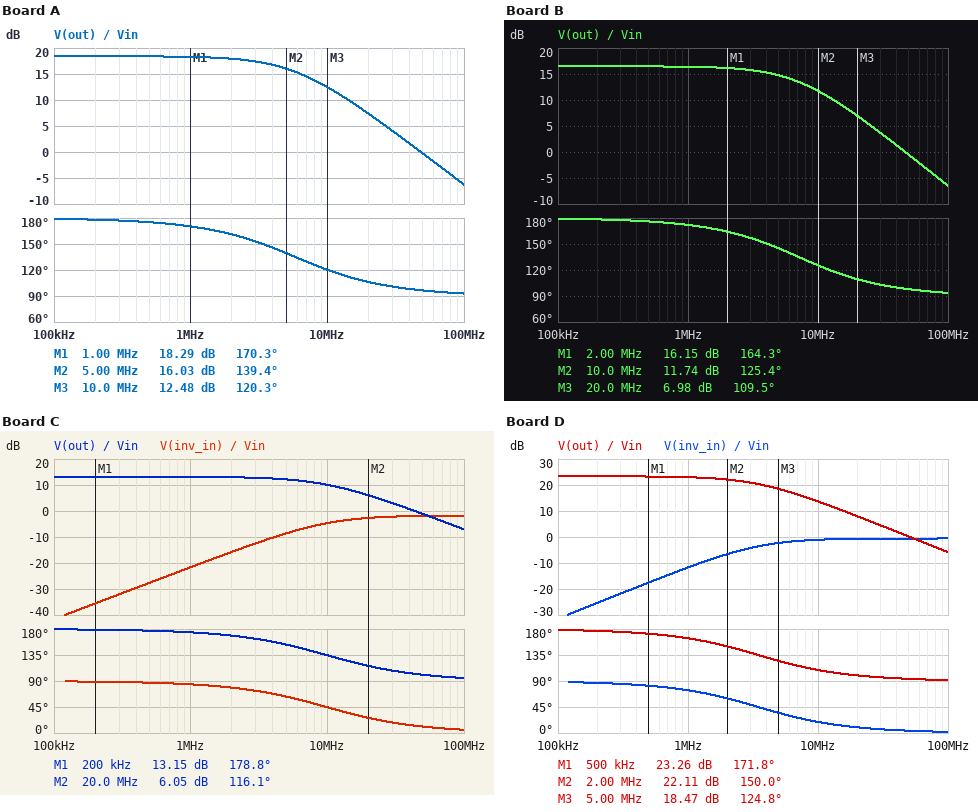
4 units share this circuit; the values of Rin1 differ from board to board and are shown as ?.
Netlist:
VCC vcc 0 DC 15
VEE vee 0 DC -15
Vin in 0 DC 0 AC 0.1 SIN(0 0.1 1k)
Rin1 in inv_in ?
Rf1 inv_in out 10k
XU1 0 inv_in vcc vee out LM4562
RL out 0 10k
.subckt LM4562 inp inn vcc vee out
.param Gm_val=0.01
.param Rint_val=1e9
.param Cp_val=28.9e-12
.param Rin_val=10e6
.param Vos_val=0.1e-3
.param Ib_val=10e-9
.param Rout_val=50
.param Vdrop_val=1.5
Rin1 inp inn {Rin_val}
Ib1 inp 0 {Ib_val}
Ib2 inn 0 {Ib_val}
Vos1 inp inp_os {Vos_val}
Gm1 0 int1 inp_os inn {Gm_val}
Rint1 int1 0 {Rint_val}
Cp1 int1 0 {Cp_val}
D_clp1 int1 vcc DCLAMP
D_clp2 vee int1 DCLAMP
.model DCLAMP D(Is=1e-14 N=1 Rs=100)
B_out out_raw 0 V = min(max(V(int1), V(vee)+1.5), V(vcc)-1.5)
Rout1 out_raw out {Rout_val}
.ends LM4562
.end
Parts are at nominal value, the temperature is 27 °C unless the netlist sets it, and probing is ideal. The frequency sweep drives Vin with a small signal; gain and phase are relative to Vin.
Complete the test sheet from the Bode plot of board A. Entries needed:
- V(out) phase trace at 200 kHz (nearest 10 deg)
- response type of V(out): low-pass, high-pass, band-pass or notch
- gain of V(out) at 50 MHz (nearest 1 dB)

180 deg
low-pass
0 dB
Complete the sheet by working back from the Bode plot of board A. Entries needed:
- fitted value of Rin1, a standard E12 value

1.2 kΩ
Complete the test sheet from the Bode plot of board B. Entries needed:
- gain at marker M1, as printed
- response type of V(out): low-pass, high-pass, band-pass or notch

16.15 dB
low-pass
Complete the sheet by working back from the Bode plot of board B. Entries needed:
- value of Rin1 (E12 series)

1.5 kΩ
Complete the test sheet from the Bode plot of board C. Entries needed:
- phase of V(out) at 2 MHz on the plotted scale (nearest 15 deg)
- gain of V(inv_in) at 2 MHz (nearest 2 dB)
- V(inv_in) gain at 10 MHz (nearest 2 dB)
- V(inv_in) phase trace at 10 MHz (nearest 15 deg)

165 deg
-16 dB
-4 dB
45 deg
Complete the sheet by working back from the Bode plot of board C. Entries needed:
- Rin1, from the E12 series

2.2 kΩ
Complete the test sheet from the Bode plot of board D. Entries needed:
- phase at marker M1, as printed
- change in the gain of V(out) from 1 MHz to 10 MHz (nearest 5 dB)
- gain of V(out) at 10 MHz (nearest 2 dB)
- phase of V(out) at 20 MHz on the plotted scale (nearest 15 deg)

171.8 deg
-10 dB
14 dB
105 deg
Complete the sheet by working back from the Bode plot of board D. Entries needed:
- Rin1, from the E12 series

680 Ω
